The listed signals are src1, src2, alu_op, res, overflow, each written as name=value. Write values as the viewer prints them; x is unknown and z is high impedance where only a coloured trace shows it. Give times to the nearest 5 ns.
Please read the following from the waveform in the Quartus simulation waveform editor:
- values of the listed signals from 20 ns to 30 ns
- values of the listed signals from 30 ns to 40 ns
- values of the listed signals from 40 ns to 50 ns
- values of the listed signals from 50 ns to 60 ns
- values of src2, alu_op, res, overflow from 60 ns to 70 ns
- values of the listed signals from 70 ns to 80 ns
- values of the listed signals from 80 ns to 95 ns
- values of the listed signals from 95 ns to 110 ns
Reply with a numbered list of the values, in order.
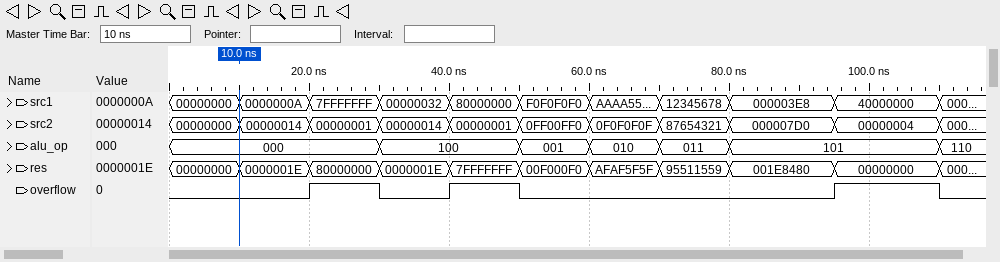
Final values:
1. src1=7FFFFFFF, src2=00000001, alu_op=000, res=80000000, overflow=1
2. src1=00000032, src2=00000014, alu_op=100, res=0000001E, overflow=0
3. src1=80000000, src2=00000001, alu_op=100, res=7FFFFFFF, overflow=1
4. src1=F0F0F0F0, src2=0FF00FF0, alu_op=001, res=00F000F0, overflow=0
5. src2=0F0F0F0F, alu_op=010, res=AFAF5F5F, overflow=0
6. src1=12345678, src2=87654321, alu_op=011, res=95511559, overflow=0
7. src1=000003E8, src2=000007D0, alu_op=101, res=001E8480, overflow=0
8. src1=40000000, src2=00000004, alu_op=101, res=00000000, overflow=1
